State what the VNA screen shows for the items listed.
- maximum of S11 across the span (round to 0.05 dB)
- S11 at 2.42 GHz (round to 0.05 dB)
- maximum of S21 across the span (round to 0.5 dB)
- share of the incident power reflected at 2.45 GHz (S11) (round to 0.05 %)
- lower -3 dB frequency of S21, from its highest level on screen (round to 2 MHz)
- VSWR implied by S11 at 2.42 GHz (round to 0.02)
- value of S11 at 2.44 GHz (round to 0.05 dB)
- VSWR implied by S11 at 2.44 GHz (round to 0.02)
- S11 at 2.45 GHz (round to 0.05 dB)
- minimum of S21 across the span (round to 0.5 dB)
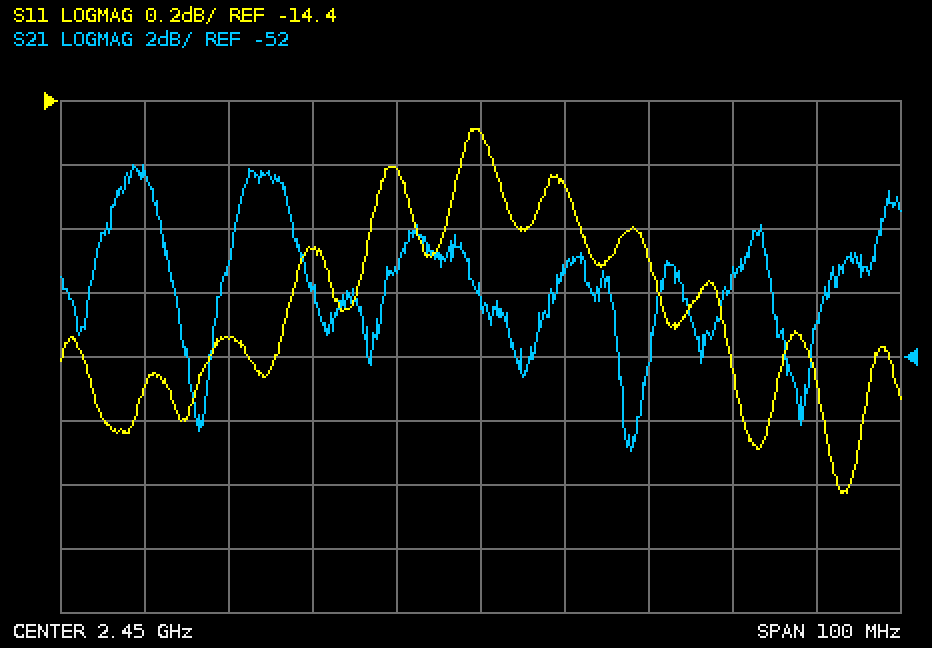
-14.50 dB
-15.15 dB
-46.0 dB
3.55 %
2.404 GHz
1.42
-14.60 dB
1.46
-14.50 dB
-55.0 dB
